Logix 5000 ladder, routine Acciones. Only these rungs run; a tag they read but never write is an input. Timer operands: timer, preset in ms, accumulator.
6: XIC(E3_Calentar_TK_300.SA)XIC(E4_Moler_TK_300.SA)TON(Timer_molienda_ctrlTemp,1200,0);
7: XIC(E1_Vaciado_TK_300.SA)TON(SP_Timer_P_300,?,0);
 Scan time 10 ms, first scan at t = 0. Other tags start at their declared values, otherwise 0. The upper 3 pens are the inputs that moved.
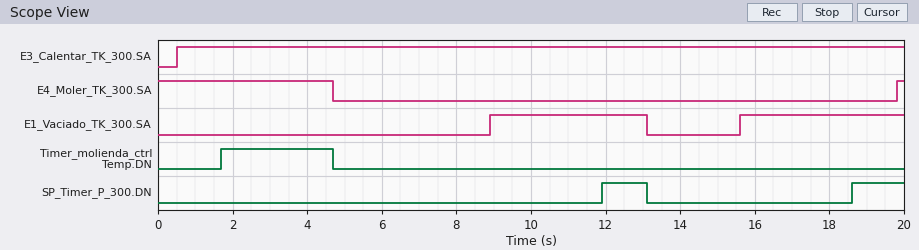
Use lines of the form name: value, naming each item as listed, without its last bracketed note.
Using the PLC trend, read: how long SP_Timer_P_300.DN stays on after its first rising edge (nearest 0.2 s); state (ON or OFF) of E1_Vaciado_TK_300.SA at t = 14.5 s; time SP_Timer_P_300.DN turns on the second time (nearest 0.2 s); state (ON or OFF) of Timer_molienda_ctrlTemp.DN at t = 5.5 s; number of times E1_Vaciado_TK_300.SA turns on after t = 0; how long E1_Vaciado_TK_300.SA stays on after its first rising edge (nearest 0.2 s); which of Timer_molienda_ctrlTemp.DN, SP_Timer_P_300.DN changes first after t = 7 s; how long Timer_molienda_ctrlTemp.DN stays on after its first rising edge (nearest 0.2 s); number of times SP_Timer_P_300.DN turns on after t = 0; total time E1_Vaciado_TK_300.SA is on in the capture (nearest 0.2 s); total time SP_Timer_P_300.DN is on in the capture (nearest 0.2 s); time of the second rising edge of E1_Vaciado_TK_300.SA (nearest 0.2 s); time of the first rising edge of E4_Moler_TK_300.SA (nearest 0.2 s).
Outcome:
how long SP_Timer_P_300.DN stays on after its first rising edge: 1.2 s
state (ON or OFF) of E1_Vaciado_TK_300.SA at t = 14.5 s: OFF
time SP_Timer_P_300.DN turns on the second time: 18.6 s
state (ON or OFF) of Timer_molienda_ctrlTemp.DN at t = 5.5 s: OFF
number of times E1_Vaciado_TK_300.SA turns on after t = 0: 2
how long E1_Vaciado_TK_300.SA stays on after its first rising edge: 4.2 s
which of Timer_molienda_ctrlTemp.DN, SP_Timer_P_300.DN changes first after t = 7 s: SP_Timer_P_300.DN
how long Timer_molienda_ctrlTemp.DN stays on after its first rising edge: 3.0 s
number of times SP_Timer_P_300.DN turns on after t = 0: 2
total time E1_Vaciado_TK_300.SA is on in the capture: 8.6 s
total time SP_Timer_P_300.DN is on in the capture: 2.6 s
time of the second rising edge of E1_Vaciado_TK_300.SA: 15.6 s
time of the first rising edge of E4_Moler_TK_300.SA: 19.8 s
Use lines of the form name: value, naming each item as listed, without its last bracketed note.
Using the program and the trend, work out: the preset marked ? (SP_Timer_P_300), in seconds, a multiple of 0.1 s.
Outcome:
the preset marked ? (SP_Timer_P_300), in seconds, a multiple of 0.1 s: 3.0 s
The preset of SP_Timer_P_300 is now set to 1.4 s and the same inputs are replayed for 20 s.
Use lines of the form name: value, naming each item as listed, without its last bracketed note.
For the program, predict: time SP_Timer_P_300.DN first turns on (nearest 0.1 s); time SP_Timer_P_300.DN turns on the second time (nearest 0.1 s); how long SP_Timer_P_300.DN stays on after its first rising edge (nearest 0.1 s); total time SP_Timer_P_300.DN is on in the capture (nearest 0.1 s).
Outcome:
time SP_Timer_P_300.DN first turns on: 10.3 s
time SP_Timer_P_300.DN turns on the second time: 17.0 s
how long SP_Timer_P_300.DN stays on after its first rising edge: 2.8 s
total time SP_Timer_P_300.DN is on in the capture: 5.8 s
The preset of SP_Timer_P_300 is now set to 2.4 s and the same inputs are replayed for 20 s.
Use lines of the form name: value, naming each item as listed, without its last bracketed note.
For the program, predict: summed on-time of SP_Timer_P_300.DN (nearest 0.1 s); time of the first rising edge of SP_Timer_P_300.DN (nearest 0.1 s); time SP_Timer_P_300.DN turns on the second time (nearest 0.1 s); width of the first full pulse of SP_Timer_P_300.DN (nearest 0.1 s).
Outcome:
summed on-time of SP_Timer_P_300.DN: 3.8 s
time of the first rising edge of SP_Timer_P_300.DN: 11.3 s
time SP_Timer_P_300.DN turns on the second time: 18.0 s
width of the first full pulse of SP_Timer_P_300.DN: 1.8 s
